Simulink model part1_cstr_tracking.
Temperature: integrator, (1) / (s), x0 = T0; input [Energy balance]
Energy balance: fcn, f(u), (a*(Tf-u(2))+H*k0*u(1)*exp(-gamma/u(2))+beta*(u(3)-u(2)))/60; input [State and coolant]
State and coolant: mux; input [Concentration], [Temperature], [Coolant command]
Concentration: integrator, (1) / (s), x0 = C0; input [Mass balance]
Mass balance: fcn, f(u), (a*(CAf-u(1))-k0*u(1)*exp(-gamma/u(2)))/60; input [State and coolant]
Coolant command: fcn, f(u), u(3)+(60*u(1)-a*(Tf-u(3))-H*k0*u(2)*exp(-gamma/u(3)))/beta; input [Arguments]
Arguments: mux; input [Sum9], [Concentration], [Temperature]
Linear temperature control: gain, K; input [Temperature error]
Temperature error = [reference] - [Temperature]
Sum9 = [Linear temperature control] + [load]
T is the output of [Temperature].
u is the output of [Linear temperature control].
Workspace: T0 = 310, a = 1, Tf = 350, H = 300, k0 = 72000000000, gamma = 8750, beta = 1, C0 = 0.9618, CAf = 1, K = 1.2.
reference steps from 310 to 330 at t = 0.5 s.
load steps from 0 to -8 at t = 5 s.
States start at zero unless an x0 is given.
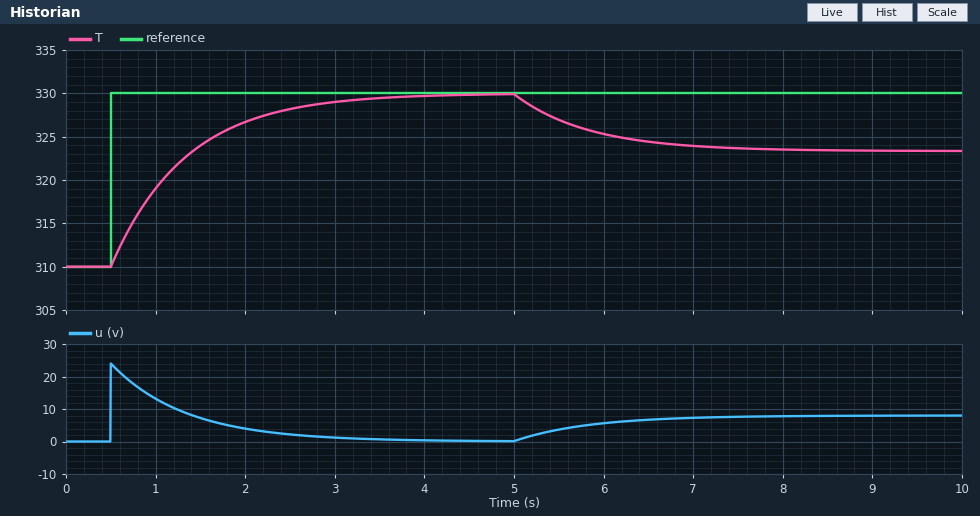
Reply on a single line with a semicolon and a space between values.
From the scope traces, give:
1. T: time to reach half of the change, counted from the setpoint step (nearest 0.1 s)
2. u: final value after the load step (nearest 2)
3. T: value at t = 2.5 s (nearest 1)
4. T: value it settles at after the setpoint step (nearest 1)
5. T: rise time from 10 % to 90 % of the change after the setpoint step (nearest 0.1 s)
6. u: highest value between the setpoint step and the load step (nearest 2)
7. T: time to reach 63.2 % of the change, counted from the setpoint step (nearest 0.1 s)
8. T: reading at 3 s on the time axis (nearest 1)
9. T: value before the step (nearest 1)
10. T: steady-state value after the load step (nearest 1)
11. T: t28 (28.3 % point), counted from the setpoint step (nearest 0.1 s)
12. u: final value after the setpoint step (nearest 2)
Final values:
0.6 s; 8; 328; 330; 1.8 s; 24; 0.8 s; 329; 310; 323; 0.3 s; 0
